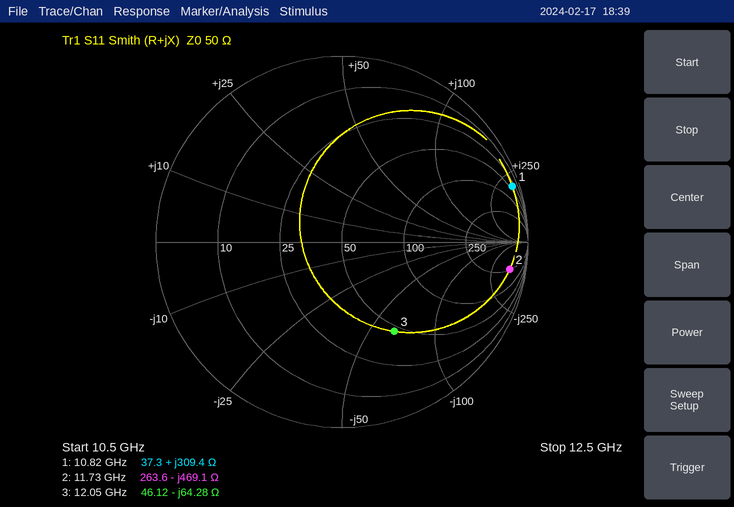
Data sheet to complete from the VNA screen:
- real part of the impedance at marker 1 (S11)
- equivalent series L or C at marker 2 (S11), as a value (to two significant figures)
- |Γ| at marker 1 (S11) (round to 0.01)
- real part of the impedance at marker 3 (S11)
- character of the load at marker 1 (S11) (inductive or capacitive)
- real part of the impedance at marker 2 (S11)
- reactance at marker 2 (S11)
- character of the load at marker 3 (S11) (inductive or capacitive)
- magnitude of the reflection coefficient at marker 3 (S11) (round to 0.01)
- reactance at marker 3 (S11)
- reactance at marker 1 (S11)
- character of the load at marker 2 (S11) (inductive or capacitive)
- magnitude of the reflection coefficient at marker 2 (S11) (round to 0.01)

37.3 Ω
29 fF
0.96
46.12 Ω
inductive
263.6 Ω
-469.1 Ω
capacitive
0.56
-64.28 Ω
+309.4 Ω
capacitive
0.91
